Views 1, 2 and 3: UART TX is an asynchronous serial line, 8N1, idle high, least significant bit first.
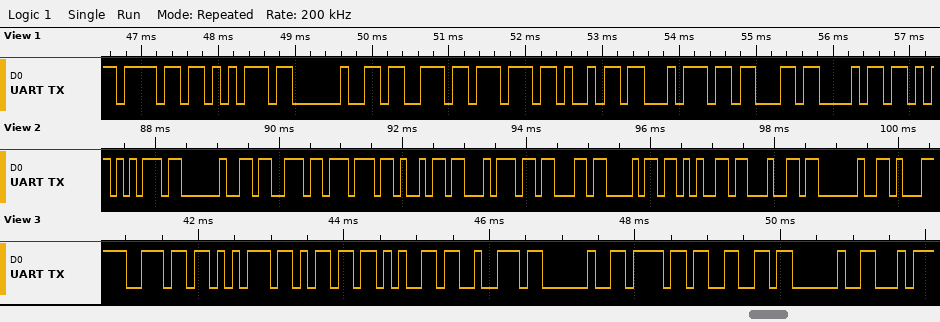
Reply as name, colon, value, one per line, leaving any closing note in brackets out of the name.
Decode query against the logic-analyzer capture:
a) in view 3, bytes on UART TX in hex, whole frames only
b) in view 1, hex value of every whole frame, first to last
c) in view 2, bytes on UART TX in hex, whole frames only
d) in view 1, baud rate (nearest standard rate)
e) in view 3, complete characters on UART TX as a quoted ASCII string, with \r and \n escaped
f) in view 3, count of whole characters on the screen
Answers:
in view 3, bytes on UART TX in hex, whole frames only: 6E 75 6D 65 72 20 6F 66 20
in view 1, hex value of every whole frame, first to last: 6F 75 20 73 77 69 74 63 68
in view 2, bytes on UART TX in hex, whole frames only: 75 20 73 77 69 74 63 68 65 64 20
in view 1, baud rate: 9600 baud
in view 3, complete characters on UART TX as a quoted ASCII string, with \r and \n escaped: "numer of "
in view 3, count of whole characters on the screen: 9
